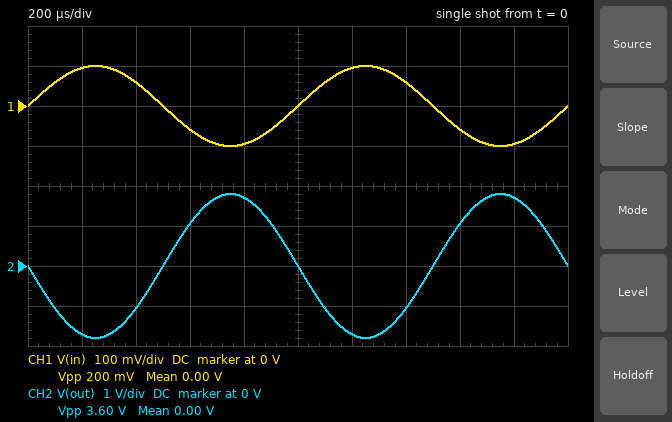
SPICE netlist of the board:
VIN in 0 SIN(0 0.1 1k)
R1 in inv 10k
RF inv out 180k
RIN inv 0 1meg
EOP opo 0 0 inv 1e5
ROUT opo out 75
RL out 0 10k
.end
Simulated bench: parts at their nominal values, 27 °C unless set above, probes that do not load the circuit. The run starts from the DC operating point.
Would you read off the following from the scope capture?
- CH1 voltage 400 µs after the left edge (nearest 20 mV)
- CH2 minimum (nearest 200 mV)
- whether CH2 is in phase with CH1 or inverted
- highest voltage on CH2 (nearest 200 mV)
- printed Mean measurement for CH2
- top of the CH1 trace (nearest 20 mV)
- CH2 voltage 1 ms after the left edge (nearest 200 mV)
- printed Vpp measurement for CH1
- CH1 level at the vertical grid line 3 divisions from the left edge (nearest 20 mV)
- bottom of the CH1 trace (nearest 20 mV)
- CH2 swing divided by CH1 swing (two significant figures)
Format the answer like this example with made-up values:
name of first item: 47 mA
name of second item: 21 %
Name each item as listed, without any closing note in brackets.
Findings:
CH1 voltage 400 µs after the left edge: 60 mV
CH2 minimum: -1.8 V
whether CH2 is in phase with CH1 or inverted: inverted
highest voltage on CH2: 1.8 V
printed Mean measurement for CH2: 0.00 V
top of the CH1 trace: 100 mV
CH2 voltage 1 ms after the left edge: 0 V
printed Vpp measurement for CH1: 200 mV
CH1 level at the vertical grid line 3 divisions from the left edge: -60 mV
bottom of the CH1 trace: -100 mV
CH2 swing divided by CH1 swing: 18
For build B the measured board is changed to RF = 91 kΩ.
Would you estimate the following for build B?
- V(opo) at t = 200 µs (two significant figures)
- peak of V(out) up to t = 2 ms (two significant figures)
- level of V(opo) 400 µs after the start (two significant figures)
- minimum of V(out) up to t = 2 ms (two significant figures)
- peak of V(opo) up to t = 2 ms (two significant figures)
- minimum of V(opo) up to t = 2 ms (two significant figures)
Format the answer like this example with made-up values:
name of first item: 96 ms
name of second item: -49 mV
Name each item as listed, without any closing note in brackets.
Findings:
V(opo) at t = 200 µs: -870 mV
peak of V(out) up to t = 2 ms: 910 mV
level of V(opo) 400 µs after the start: -540 mV
minimum of V(out) up to t = 2 ms: -910 mV
peak of V(opo) up to t = 2 ms: 920 mV
minimum of V(opo) up to t = 2 ms: -920 mV
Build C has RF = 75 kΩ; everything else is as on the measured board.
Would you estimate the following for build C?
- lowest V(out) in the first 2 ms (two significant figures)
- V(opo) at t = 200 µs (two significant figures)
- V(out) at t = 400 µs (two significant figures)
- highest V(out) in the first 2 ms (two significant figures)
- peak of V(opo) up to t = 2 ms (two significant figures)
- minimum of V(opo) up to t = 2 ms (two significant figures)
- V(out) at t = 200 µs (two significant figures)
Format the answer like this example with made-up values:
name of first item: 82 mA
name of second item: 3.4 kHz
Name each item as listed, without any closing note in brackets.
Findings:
lowest V(out) in the first 2 ms: -750 mV
V(opo) at t = 200 µs: -720 mV
V(out) at t = 400 µs: -440 mV
highest V(out) in the first 2 ms: 750 mV
peak of V(opo) up to t = 2 ms: 760 mV
minimum of V(opo) up to t = 2 ms: -760 mV
V(out) at t = 200 µs: -710 mV
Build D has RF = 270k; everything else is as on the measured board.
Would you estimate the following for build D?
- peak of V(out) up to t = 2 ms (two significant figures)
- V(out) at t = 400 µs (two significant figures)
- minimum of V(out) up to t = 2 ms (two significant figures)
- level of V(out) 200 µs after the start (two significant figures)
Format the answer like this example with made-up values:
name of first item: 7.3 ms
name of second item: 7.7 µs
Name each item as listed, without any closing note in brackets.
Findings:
peak of V(out) up to t = 2 ms: 2.7 V
V(out) at t = 400 µs: -1.6 V
minimum of V(out) up to t = 2 ms: -2.7 V
level of V(out) 200 µs after the start: -2.6 V
